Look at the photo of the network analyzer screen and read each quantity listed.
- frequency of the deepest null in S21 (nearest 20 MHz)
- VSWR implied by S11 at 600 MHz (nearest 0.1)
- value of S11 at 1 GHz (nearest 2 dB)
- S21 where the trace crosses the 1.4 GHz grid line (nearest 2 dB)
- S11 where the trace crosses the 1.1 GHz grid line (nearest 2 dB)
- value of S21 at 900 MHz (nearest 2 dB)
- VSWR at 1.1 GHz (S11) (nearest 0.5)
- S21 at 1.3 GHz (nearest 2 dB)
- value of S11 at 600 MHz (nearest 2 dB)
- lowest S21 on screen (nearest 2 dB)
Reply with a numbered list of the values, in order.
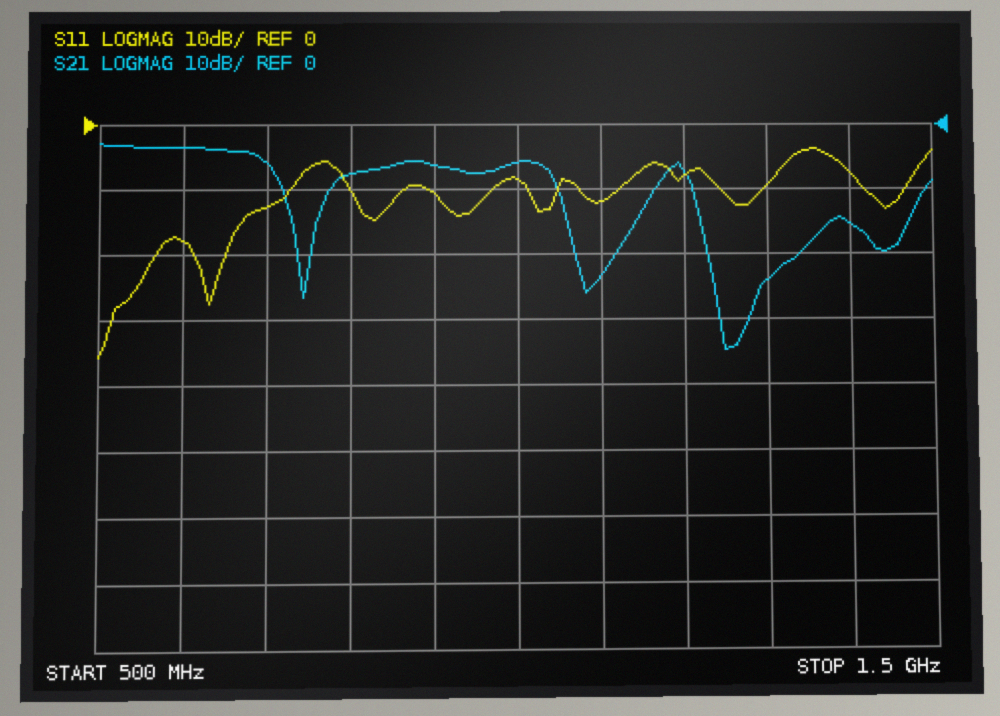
1. 1.24 GHz
2. 1.3
3. -8 dB
4. -16 dB
5. -12 dB
6. -6 dB
7. 1.5
8. -24 dB
9. -18 dB
10. -34 dB
